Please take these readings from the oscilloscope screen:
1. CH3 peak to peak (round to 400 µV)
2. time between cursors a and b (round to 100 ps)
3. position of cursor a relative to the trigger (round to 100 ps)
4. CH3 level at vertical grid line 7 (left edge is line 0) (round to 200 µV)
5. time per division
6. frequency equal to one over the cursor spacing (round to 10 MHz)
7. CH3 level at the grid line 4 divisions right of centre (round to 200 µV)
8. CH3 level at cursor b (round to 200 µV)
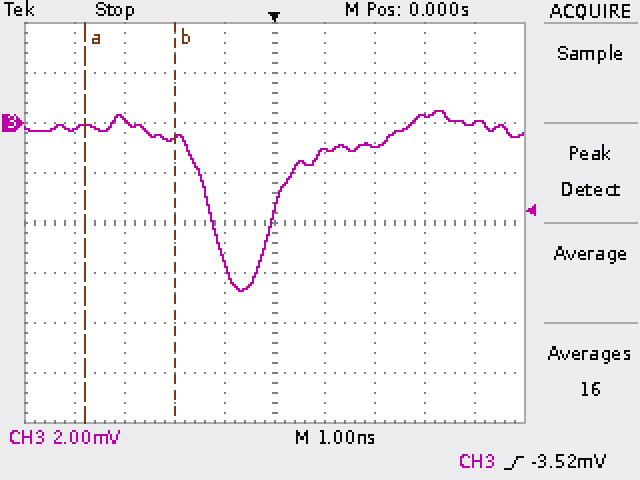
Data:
7.2 mV
1.8 ns
-3.8 ns
-1.0 mV
1 ns
560 MHz
0.0 mV
-600 µV
